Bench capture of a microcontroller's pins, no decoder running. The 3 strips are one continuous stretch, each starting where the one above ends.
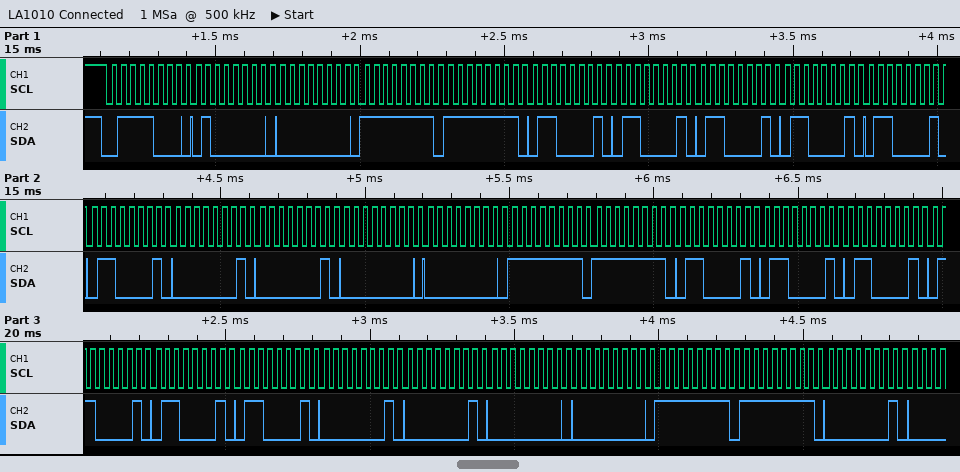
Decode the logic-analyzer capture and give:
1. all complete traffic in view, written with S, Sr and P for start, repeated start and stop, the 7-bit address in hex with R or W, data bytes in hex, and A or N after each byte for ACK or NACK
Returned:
S 3CW A 40 A 00 A FF A FF A 61 A 61 A 61 A 61 A 61 A 61 A 01 A 01 A 00 A 00 A FF A FF A 61 A 61 A 61 A 61 A 61 A 61 A 01 A 01 A 00 A 00 A FF A FF A 01 A
